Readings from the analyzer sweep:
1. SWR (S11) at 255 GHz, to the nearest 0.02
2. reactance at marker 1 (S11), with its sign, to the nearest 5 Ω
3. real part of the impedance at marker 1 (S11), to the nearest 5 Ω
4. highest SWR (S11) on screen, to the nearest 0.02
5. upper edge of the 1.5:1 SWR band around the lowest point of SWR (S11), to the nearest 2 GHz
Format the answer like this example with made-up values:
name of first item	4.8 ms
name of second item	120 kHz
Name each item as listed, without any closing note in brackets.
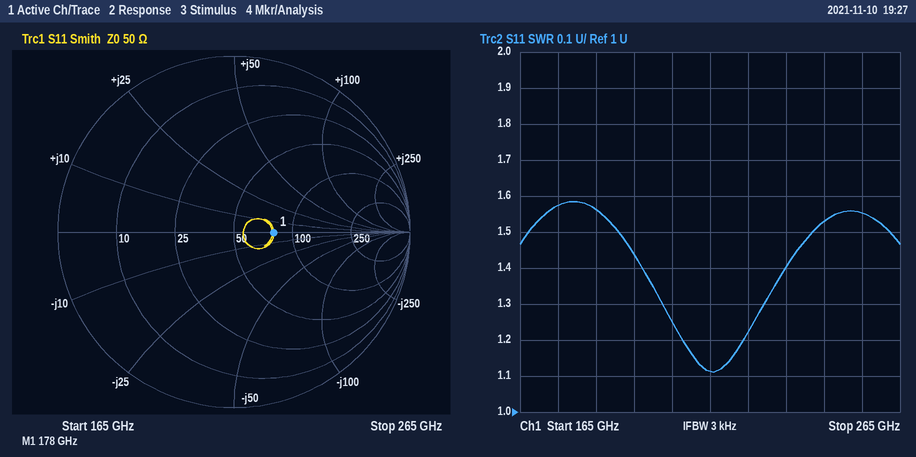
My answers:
SWR (S11) at 255 GHz, to the nearest 0.02	1.56
reactance at marker 1 (S11), with its sign, to the nearest 5 Ω	0 Ω
real part of the impedance at marker 1 (S11), to the nearest 5 Ω	80 Ω
highest SWR (S11) on screen, to the nearest 0.02	1.58
upper edge of the 1.5:1 SWR band around the lowest point of SWR (S11), to the nearest 2 GHz	242 GHz
